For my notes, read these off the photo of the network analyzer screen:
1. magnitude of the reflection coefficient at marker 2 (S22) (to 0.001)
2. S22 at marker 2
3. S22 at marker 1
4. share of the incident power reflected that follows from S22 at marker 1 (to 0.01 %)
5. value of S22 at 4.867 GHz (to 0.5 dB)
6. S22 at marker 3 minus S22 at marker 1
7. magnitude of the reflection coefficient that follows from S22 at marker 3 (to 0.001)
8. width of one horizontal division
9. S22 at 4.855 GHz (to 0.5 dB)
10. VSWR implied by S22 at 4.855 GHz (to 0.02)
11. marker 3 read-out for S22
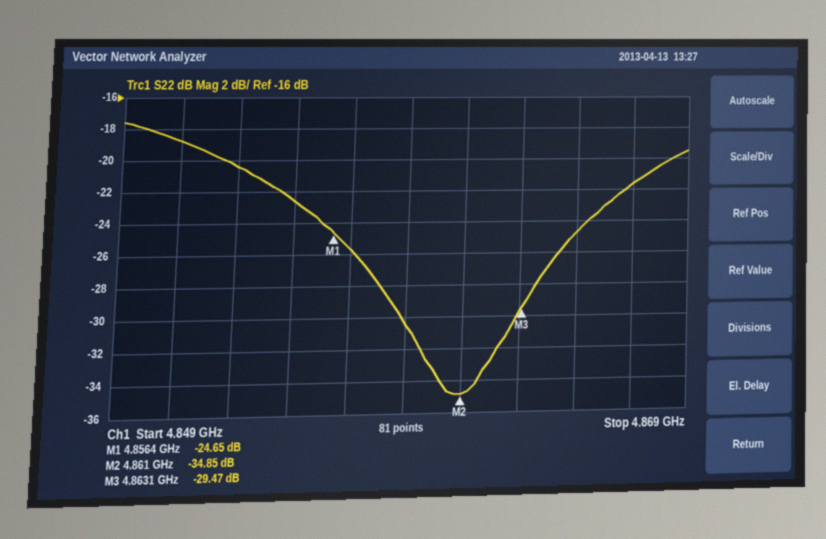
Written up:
0.018
-34.85 dB
-24.65 dB
0.34 %
-21.5 dB
-4.82 dB
0.034
2 MHz
-22.5 dB
1.16
-29.47 dB
